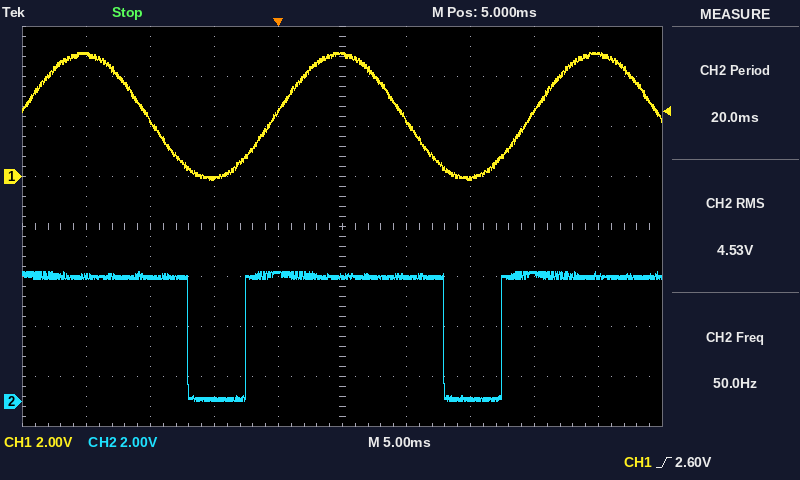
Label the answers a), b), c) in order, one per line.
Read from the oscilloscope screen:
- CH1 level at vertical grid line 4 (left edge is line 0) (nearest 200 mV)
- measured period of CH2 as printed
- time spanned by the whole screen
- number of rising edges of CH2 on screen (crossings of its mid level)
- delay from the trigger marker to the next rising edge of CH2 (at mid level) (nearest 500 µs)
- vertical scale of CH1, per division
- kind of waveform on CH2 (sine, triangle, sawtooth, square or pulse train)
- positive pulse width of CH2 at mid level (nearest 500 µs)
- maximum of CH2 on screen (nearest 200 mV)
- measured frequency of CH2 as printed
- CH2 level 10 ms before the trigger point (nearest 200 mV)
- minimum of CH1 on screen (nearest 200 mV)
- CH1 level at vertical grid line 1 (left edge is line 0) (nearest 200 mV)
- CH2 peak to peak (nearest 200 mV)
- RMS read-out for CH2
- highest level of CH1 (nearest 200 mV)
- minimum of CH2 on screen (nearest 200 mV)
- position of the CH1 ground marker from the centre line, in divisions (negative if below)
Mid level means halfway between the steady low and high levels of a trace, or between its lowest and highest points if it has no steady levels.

a) 2.6 V
b) 20.0 ms
c) 50 ms
d) 2
e) 17.5 ms
f) 2 V
g) pulse train
h) 15.5 ms
i) 5.2 V
j) 50.0 Hz
k) 5.0 V
l) -200 mV
m) 4.8 V
n) 5.2 V
o) 4.53 V
p) 5.0 V
q) 0.0 V
r) +1.0 div
